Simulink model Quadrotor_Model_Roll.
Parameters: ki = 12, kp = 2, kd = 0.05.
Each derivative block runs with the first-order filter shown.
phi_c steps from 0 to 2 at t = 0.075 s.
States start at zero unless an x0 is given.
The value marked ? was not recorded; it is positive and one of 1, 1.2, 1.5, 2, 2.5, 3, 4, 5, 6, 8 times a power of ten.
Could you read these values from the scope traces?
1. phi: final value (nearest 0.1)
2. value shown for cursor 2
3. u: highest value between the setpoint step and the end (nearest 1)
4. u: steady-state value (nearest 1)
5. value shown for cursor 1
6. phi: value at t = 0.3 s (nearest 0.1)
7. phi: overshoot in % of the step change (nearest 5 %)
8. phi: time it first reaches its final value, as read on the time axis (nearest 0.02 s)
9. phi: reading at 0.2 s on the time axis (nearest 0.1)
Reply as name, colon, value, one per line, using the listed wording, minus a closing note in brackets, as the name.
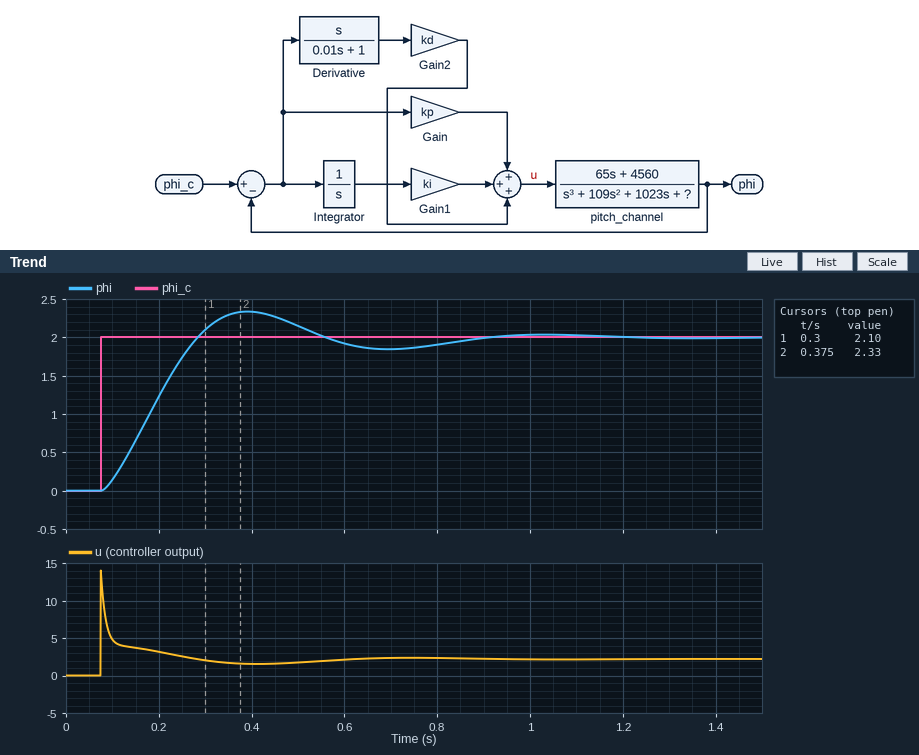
phi: final value: 2.0
value shown for cursor 2: 2.33
u: highest value between the setpoint step and the end: 14
u: steady-state value: 2
value shown for cursor 1: 2.10
phi: value at t = 0.3 s: 2.1
phi: overshoot in % of the step change: 15 %
phi: time it first reaches its final value, as read on the time axis: 0.28 s
phi: reading at 0.2 s on the time axis: 1.2
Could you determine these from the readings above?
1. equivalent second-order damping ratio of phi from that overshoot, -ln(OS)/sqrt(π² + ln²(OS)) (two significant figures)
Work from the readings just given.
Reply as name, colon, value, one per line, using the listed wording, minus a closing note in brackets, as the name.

equivalent second-order damping ratio of phi from that overshoot, -ln(OS)/sqrt(π² + ln²(OS)): 0.52
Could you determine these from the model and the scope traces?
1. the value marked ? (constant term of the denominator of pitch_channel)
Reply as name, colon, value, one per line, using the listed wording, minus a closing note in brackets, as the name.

the value marked ?: 5000
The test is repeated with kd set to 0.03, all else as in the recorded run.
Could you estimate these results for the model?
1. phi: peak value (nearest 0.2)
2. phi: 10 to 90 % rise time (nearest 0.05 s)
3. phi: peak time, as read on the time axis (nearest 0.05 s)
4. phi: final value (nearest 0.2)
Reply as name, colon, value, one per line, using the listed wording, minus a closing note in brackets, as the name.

phi: peak value: 2.4
phi: 10 to 90 % rise time: 0.15 s
phi: peak time, as read on the time axis: 0.40 s
phi: final value: 2.0
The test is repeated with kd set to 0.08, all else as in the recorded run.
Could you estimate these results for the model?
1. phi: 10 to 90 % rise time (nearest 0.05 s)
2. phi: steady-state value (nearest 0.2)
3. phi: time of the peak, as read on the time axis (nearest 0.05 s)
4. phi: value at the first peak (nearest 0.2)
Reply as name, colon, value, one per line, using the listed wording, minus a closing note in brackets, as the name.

phi: 10 to 90 % rise time: 0.15 s
phi: steady-state value: 2.0
phi: time of the peak, as read on the time axis: 0.40 s
phi: value at the first peak: 2.2
